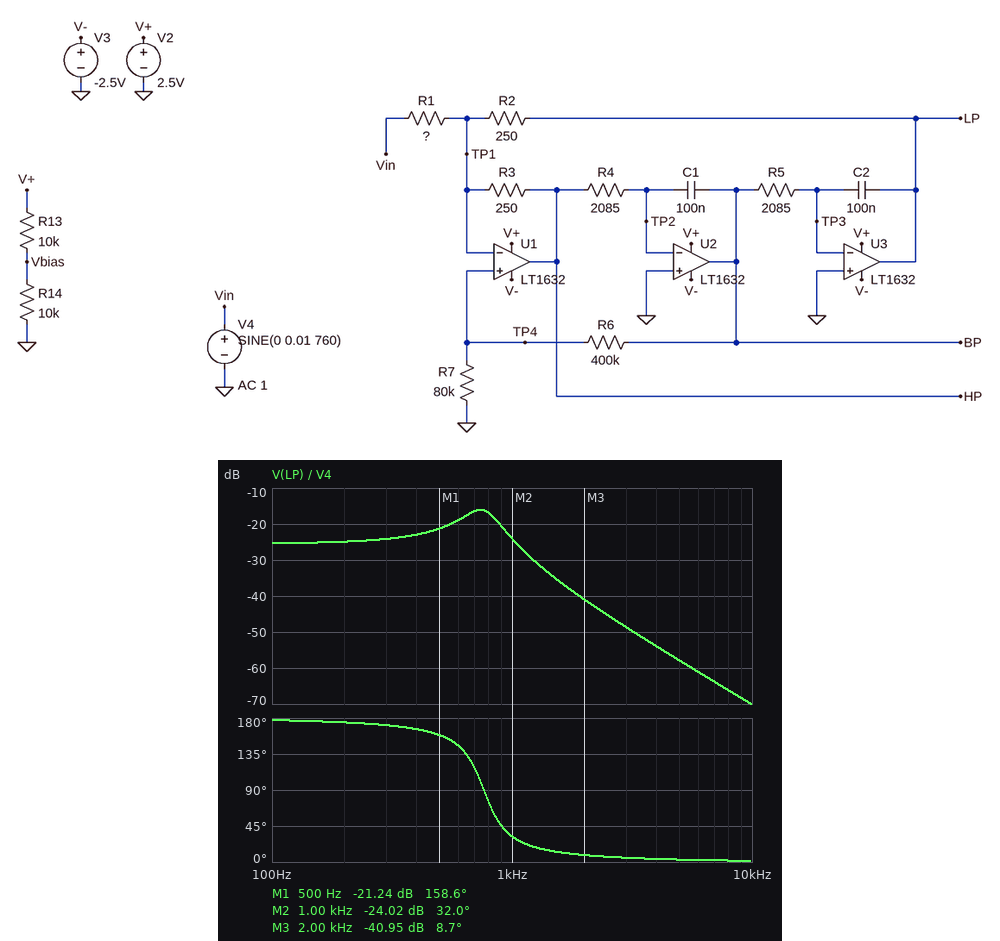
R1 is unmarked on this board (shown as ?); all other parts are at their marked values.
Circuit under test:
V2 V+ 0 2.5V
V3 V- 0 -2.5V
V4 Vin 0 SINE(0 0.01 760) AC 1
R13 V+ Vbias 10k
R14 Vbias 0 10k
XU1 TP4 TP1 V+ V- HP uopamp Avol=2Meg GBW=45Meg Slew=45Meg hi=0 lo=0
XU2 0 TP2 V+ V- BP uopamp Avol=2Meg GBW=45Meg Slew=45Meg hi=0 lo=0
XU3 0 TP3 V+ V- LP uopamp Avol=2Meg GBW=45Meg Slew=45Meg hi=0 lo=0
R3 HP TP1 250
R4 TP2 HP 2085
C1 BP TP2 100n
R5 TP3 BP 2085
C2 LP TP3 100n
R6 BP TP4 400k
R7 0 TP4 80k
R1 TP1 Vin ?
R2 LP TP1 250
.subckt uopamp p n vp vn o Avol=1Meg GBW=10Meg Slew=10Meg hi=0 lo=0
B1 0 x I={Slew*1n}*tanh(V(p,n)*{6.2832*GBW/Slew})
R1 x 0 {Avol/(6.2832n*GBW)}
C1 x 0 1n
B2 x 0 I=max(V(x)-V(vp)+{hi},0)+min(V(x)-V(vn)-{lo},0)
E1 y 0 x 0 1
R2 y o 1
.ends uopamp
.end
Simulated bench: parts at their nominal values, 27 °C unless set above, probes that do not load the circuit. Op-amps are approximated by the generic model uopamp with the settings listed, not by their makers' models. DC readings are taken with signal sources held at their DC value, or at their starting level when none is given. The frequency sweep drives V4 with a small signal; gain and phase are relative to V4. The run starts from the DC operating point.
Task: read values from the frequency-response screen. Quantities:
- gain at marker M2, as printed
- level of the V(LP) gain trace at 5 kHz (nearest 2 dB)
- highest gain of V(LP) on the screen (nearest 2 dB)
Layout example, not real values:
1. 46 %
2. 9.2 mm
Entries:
1. -24.02 dB
2. -58 dB
3. -16 dB
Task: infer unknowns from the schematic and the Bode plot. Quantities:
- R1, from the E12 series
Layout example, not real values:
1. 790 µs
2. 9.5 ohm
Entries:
1. 4.7 kΩ
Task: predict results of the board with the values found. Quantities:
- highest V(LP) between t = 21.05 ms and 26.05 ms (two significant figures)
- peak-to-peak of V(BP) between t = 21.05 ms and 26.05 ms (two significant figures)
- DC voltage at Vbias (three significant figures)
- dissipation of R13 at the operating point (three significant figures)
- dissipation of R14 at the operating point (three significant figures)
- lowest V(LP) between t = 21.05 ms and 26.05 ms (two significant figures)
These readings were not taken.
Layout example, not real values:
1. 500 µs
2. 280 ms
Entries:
1. 1.6 mV
2. 3.1 mV
3. 1.25 V
4. 156 µW
5. 156 µW
6. -1.6 mV
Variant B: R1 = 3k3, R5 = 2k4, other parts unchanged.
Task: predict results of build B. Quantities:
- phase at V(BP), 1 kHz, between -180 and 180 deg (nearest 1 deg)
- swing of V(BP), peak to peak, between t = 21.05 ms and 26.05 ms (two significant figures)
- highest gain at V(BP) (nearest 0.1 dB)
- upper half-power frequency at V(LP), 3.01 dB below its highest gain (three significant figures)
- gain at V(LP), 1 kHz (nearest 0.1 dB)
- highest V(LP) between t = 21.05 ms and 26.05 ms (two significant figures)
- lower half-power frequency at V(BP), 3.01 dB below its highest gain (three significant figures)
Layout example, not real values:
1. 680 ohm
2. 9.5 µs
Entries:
1. -62 deg
2. 4.1 mV
3. -13.2 dB
4. 810 Hz
5. -23.3 dB
6. 1.8 mV
7. 592 Hz
